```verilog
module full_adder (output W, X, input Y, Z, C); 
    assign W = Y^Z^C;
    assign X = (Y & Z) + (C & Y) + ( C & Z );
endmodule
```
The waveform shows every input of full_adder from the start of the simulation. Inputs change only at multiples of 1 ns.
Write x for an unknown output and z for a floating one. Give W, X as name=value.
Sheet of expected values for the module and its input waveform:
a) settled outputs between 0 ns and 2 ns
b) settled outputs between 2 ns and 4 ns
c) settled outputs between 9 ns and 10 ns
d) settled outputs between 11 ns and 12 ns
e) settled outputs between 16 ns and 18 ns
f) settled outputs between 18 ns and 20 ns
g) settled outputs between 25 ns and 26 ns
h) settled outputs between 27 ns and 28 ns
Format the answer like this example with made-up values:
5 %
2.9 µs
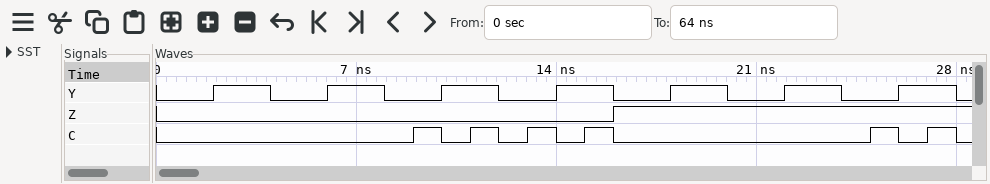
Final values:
W=0, X=0
W=1, X=0
W=1, X=0
W=0, X=1
W=1, X=0
W=0, X=1
W=0, X=1
W=1, X=1
